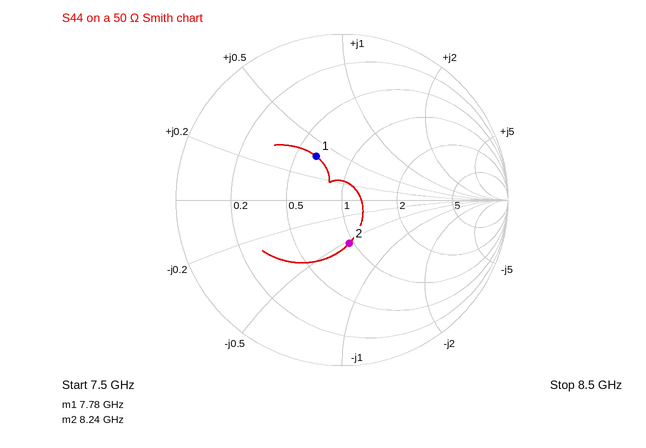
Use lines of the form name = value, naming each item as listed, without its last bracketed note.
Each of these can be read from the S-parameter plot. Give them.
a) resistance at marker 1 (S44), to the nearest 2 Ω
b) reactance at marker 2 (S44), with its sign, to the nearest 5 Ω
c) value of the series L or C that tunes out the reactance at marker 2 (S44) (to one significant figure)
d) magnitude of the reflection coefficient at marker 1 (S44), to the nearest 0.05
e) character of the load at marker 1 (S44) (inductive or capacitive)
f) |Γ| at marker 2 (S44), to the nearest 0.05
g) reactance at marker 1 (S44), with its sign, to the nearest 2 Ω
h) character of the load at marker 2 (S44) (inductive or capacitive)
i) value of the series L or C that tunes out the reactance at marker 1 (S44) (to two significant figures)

resistance at marker 1 (S44), to the nearest 2 Ω = 32 Ω
reactance at marker 2 (S44), with its sign, to the nearest 5 Ω = -25 Ω
value of the series L or C that tunes out the reactance at marker 2 (S44) = 500 pH
magnitude of the reflection coefficient at marker 1 (S44), to the nearest 0.05 = 0.30
character of the load at marker 1 (S44) = inductive
|Γ| at marker 2 (S44), to the nearest 0.05 = 0.25
reactance at marker 1 (S44), with its sign, to the nearest 2 Ω = +18 Ω
character of the load at marker 2 (S44) = capacitive
value of the series L or C that tunes out the reactance at marker 1 (S44) = 1.1 pF
